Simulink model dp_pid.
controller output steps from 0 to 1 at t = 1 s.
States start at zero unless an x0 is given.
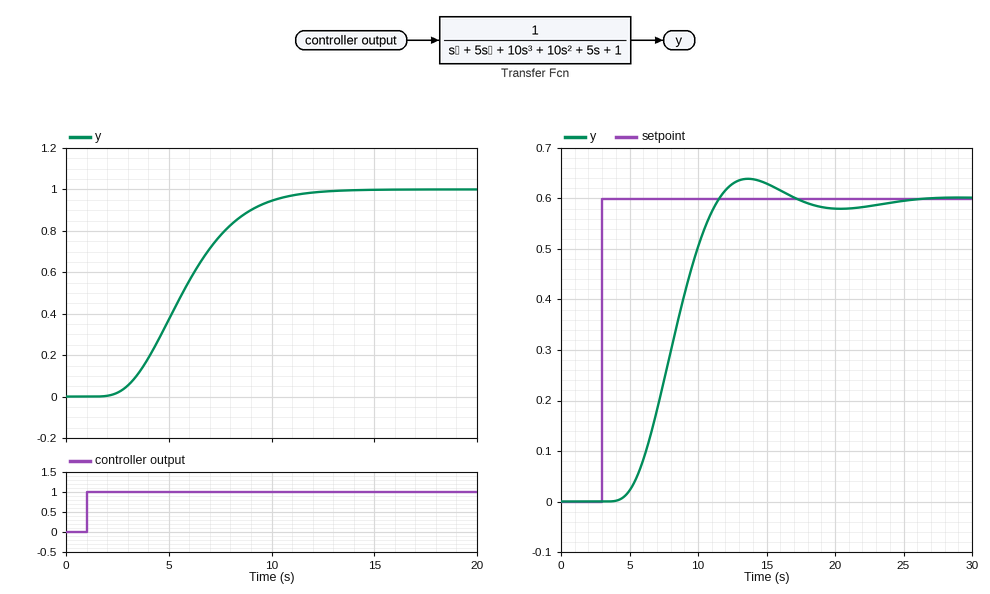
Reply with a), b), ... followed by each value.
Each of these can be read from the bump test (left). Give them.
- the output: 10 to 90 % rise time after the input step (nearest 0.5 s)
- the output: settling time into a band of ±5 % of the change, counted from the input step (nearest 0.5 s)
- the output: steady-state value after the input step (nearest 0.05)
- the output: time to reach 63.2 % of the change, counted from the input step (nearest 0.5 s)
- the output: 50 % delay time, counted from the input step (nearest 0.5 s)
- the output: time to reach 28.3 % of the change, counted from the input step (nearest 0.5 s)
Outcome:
a) 5.5 s
b) 9.0 s
c) 1.00
d) 5.5 s
e) 4.5 s
f) 3.5 s
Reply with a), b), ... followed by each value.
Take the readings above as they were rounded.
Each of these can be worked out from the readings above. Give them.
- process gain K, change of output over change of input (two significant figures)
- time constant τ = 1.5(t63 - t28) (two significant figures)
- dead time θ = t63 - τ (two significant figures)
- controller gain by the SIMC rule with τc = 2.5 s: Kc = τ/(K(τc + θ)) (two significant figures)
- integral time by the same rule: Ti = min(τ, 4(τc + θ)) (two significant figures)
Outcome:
a) 1.0
b) 3.0 s
c) 2.5 s
d) 0.60
e) 3.0 s
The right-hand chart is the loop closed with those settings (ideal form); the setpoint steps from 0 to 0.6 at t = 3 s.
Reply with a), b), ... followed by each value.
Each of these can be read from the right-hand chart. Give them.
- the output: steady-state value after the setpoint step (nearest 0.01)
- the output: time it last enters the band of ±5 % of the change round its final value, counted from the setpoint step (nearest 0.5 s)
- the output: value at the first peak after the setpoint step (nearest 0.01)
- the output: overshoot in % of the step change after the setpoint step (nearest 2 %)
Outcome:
a) 0.60
b) 12.0 s
c) 0.64
d) 6 %
